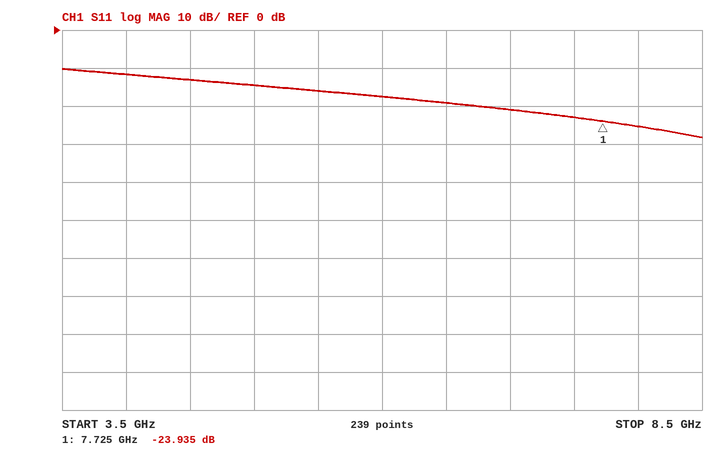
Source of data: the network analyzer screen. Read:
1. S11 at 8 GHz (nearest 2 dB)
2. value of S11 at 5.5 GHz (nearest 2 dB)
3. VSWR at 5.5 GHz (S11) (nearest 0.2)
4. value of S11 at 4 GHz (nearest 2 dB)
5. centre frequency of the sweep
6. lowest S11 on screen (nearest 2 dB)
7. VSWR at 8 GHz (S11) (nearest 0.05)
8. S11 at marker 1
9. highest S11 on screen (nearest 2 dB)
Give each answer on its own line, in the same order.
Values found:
-26 dB
-16 dB
1.4
-12 dB
6 GHz
-28 dB
1.10
-23.935 dB
-10 dB
